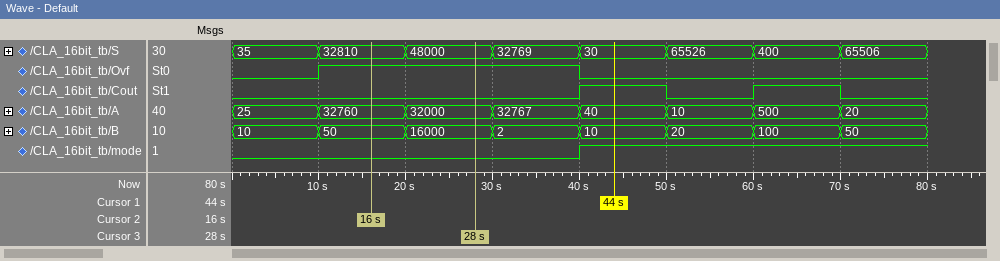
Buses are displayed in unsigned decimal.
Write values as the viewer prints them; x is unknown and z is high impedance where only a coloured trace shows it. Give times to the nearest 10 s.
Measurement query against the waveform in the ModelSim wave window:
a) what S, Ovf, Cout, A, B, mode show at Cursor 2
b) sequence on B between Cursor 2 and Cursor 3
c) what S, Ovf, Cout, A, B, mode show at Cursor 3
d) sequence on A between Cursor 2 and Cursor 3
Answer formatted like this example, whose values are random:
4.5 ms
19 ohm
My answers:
S=32810, Ovf=1, Cout=0, A=32760, B=50, mode=0
50, 16000
S=48000, Ovf=1, Cout=0, A=32000, B=16000, mode=0
32760, 32000
